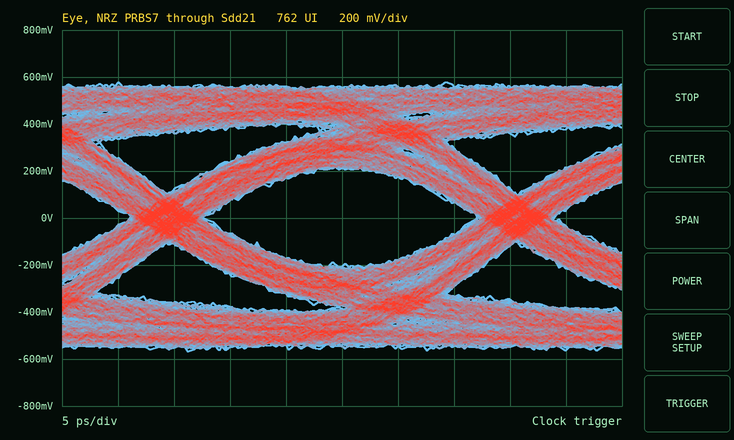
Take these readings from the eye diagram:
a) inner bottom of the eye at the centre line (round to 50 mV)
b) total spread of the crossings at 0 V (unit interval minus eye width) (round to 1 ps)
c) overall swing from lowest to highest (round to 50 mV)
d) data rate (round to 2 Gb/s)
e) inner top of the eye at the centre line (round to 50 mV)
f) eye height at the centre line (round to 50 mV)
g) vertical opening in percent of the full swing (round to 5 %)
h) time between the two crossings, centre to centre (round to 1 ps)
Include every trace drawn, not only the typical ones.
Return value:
-200 mV
7 ps
1.15 V
32 Gb/s
200 mV
400 mV
35 %
31 ps
